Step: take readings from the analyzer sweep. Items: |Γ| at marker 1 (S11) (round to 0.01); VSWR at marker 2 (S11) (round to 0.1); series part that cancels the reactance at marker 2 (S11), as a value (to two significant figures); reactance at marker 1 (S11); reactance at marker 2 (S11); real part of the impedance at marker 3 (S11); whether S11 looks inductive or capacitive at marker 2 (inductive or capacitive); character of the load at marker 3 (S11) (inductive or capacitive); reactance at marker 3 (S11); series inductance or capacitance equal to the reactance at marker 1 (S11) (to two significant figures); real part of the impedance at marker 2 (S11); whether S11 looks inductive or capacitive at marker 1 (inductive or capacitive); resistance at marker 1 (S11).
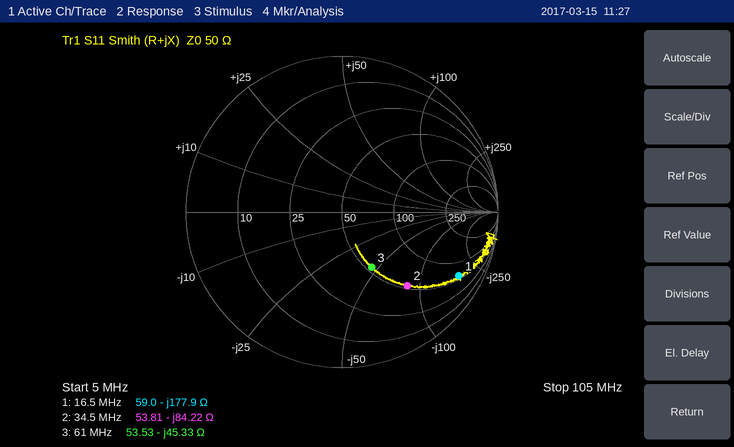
0.85
4.4
390 nH
-177.9 Ω
-84.22 Ω
53.53 Ω
capacitive
capacitive
-45.33 Ω
54 pF
53.81 Ω
capacitive
59.0 Ω
